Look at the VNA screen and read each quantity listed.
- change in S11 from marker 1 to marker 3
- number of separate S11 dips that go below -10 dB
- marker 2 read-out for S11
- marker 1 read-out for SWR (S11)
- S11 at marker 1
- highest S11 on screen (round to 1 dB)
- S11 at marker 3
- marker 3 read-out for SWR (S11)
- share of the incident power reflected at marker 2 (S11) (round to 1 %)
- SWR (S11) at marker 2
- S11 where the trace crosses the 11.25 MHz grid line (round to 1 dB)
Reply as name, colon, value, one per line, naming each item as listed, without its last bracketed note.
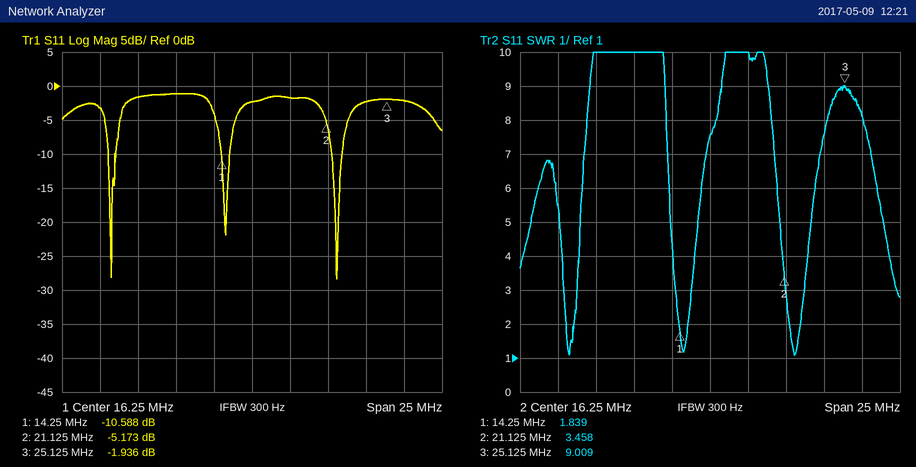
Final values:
change in S11 from marker 1 to marker 3: 8.652 dB
number of separate S11 dips that go below -10 dB: 3
marker 2 read-out for S11: -5.173 dB
marker 1 read-out for SWR: 1.839
S11 at marker 1: -10.588 dB
highest S11 on screen: -1 dB
S11 at marker 3: -1.936 dB
marker 3 read-out for SWR: 9.009
share of the incident power reflected at marker 2 (S11): 30 %
SWR (S11) at marker 2: 3.458
S11 where the trace crosses the 11.25 MHz grid line: -1 dB
